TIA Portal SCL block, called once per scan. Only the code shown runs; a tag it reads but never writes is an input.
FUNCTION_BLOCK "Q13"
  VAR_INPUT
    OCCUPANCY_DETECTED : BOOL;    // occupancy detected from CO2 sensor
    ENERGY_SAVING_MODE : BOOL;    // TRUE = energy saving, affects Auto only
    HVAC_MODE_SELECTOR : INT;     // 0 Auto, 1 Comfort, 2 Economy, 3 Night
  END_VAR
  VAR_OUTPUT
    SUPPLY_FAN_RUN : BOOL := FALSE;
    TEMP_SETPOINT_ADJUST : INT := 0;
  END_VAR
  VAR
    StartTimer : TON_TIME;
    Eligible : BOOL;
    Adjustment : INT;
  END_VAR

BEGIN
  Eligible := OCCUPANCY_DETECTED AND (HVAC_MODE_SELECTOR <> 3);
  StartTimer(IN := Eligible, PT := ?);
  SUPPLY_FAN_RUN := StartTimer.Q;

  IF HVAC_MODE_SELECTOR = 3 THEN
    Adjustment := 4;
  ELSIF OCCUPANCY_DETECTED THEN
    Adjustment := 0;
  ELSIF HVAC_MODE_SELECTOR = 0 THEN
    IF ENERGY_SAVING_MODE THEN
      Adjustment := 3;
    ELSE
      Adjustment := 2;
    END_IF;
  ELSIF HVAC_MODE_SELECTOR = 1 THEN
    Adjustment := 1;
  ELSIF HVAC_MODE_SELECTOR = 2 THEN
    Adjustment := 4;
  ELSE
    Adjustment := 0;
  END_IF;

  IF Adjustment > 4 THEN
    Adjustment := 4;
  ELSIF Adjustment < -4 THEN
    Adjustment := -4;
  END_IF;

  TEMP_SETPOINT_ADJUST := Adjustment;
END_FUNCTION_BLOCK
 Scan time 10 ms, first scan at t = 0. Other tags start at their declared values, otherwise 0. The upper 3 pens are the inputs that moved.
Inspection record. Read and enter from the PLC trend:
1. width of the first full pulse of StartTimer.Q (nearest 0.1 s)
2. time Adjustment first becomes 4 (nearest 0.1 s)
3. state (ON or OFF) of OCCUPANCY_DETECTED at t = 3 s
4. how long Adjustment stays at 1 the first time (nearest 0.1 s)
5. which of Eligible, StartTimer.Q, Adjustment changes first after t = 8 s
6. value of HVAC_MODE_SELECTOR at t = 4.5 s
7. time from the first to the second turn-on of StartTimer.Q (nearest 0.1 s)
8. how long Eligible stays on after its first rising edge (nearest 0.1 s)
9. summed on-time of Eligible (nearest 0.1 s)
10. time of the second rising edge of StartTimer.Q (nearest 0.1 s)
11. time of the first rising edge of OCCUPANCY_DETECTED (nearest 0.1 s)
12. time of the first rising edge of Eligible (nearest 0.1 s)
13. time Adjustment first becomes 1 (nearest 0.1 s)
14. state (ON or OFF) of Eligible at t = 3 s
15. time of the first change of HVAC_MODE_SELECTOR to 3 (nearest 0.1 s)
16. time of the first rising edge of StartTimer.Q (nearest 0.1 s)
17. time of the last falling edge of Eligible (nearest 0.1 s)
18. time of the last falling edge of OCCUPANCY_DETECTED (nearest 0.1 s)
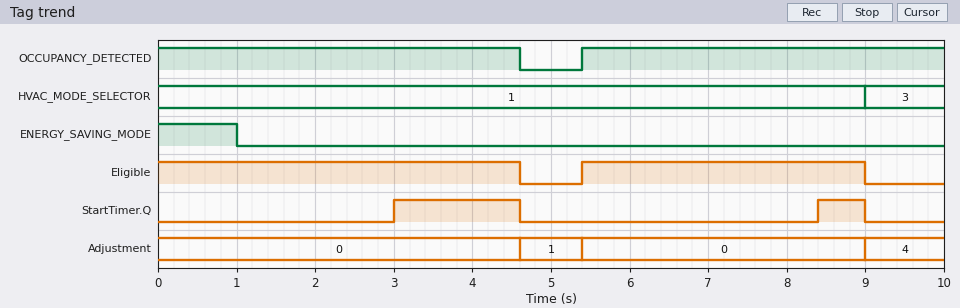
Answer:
1.6 s
9.0 s
ON
0.8 s
StartTimer.Q
1
5.4 s
3.6 s
8.2 s
8.4 s
5.4 s
5.4 s
4.6 s
ON
9.0 s
3.0 s
9.0 s
4.6 s
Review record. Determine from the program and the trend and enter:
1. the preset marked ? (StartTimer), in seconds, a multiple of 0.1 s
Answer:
3.0 s
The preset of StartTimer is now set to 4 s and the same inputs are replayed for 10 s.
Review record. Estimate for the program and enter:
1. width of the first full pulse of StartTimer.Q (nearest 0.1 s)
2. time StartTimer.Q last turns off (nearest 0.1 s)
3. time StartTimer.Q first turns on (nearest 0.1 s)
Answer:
0.6 s
4.6 s
4.0 s
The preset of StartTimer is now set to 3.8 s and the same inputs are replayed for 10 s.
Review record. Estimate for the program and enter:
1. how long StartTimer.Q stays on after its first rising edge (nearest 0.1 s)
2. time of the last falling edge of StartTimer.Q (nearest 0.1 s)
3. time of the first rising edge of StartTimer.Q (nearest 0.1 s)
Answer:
0.8 s
4.6 s
3.8 s
